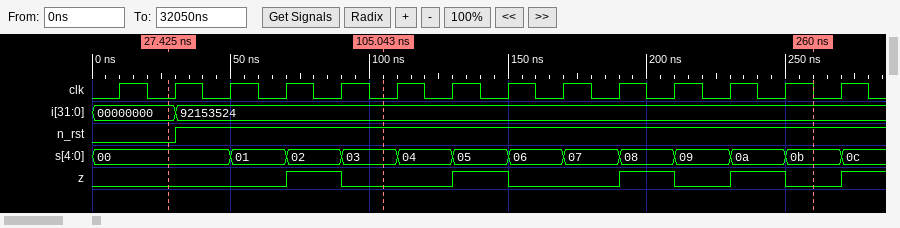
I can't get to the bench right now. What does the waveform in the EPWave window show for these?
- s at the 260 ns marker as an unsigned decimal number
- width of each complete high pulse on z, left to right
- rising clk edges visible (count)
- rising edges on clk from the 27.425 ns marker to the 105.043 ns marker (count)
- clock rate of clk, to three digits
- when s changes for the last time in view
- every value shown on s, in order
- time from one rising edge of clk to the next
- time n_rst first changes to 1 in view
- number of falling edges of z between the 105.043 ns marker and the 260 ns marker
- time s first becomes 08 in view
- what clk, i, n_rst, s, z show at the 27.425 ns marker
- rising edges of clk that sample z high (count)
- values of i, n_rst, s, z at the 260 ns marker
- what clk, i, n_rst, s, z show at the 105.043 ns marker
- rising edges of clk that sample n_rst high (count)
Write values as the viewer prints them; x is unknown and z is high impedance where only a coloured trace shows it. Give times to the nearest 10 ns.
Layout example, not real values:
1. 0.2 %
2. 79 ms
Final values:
1. 11
2. 20 ns, 20 ns, 20 ns, 20 ns
3. 14
4. 4
5. 50.0 MHz
6. 270 ns
7. 00, 01, 02, 03, 04, 05, 06, 07, 08, 09, 0a, 0b, 0c
8. 20 ns
9. 30 ns
10. 3
11. 190 ns
12. clk=0, i=00000000, n_rst=0, s=00, z=0
13. 4
14. i=92153524, n_rst=1, s=0b, z=0
15. clk=0, i=92153524, n_rst=1, s=03, z=0
16. 12
